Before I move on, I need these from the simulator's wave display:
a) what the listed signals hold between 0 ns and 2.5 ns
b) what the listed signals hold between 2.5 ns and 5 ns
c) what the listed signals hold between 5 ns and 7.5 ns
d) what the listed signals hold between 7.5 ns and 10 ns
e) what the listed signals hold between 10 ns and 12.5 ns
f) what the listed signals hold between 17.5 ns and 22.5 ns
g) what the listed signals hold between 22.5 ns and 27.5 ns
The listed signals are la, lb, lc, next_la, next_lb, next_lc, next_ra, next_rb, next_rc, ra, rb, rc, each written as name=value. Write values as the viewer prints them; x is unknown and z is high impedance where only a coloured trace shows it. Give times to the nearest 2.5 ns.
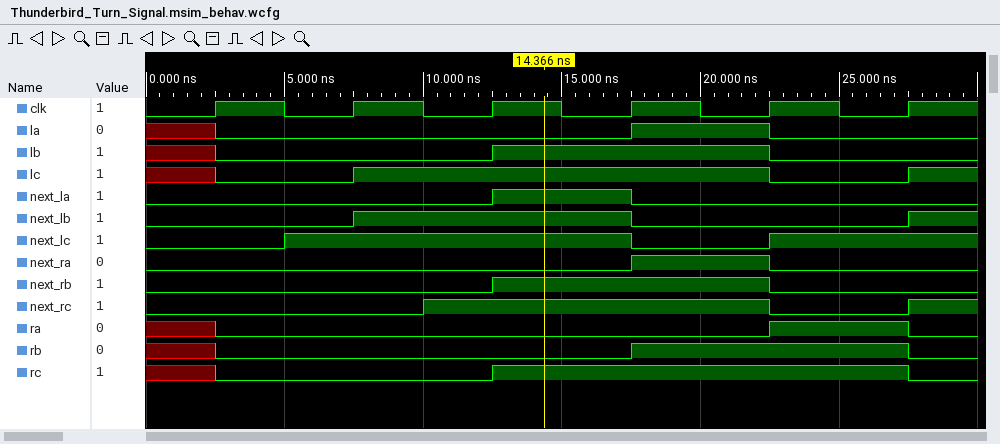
la=x, lb=x, lc=x, next_la=0, next_lb=0, next_lc=0, next_ra=0, next_rb=0, next_rc=0, ra=x, rb=x, rc=x
la=0, lb=0, lc=0, next_la=0, next_lb=0, next_lc=0, next_ra=0, next_rb=0, next_rc=0, ra=0, rb=0, rc=0
la=0, lb=0, lc=0, next_la=0, next_lb=0, next_lc=1, next_ra=0, next_rb=0, next_rc=0, ra=0, rb=0, rc=0
la=0, lb=0, lc=1, next_la=0, next_lb=1, next_lc=1, next_ra=0, next_rb=0, next_rc=0, ra=0, rb=0, rc=0
la=0, lb=0, lc=1, next_la=0, next_lb=1, next_lc=1, next_ra=0, next_rb=0, next_rc=1, ra=0, rb=0, rc=0
la=1, lb=1, lc=1, next_la=0, next_lb=0, next_lc=0, next_ra=1, next_rb=1, next_rc=1, ra=0, rb=1, rc=1
la=0, lb=0, lc=0, next_la=0, next_lb=0, next_lc=1, next_ra=0, next_rb=0, next_rc=0, ra=1, rb=1, rc=1
